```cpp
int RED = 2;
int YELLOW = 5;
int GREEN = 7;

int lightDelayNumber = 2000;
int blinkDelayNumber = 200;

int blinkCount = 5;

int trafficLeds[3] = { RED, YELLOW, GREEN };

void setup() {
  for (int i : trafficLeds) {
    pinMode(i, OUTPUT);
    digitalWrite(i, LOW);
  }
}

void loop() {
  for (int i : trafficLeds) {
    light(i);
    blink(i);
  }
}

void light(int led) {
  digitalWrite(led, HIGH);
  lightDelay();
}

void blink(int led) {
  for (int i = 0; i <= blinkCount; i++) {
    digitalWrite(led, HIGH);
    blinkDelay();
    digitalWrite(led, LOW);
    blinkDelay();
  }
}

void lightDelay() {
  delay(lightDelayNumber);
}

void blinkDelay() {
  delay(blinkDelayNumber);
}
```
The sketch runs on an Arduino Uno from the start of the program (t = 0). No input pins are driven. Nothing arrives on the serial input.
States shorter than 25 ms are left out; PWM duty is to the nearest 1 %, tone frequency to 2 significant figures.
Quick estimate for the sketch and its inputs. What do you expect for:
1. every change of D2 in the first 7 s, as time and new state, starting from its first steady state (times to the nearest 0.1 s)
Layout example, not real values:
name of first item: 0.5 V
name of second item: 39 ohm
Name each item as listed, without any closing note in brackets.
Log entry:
every change of D2 in the first 7 s, as time and new state, starting from its first steady state: 0 s high; 2.2 s low; 2.4 s high; 2.6 s low; 2.8 s high; 3 s low; 3.2 s high; 3.4 s low; 3.6 s high; 3.8 s low; 4 s high; 4.2 s low
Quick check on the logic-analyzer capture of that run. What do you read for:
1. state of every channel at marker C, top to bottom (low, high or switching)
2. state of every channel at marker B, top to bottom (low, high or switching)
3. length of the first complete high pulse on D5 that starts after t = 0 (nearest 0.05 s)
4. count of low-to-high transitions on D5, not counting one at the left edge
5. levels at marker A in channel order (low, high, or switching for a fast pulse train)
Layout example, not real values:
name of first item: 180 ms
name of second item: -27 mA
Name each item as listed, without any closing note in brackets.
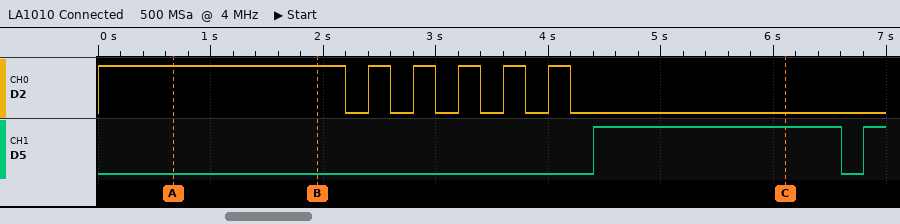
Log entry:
state of every channel at marker C, top to bottom: D2 low, D5 high
state of every channel at marker B, top to bottom: D2 high, D5 low
length of the first complete high pulse on D5 that starts after t = 0: 2.20 s
count of low-to-high transitions on D5, not counting one at the left edge: 2
levels at marker A in channel order: D2 high, D5 low
